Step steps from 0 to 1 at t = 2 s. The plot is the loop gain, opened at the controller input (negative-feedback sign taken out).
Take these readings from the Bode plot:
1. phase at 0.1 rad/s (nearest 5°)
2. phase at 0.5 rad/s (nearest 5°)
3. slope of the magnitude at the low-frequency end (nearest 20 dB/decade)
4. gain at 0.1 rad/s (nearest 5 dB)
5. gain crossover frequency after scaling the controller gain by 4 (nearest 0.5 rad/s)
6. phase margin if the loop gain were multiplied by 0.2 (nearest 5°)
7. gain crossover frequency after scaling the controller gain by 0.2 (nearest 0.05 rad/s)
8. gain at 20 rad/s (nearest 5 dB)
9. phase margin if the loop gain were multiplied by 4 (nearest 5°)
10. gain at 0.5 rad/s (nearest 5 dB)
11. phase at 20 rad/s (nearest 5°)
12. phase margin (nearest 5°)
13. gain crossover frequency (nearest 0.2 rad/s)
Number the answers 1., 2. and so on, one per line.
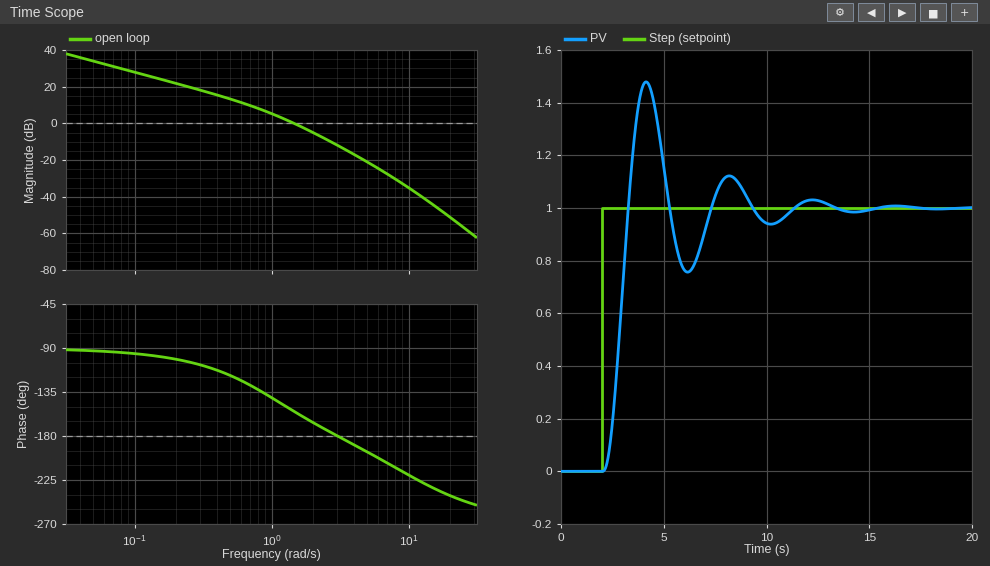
1. -95°
2. -120°
3. -20 dB/decade
4. 30 dB
5. 3.0 rad/s
6. 65°
7. 0.45 rad/s
8. -50 dB
9. 0°
10. 15 dB
11. -240°
12. 25°
13. 1.4 rad/s
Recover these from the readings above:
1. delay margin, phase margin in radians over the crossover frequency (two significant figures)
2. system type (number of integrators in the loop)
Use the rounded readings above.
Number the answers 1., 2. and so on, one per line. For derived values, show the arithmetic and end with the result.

1. 25 × π / 180 / 1.4 = 0.31 s
2. 1
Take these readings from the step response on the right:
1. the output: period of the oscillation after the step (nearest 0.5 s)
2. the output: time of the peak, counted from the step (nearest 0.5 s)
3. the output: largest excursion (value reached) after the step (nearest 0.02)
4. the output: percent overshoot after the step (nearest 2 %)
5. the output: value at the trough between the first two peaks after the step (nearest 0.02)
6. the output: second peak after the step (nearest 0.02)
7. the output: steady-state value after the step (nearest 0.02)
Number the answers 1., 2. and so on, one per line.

1. 4.0 s
2. 2.0 s
3. 1.48
4. 48 %
5. 0.76
6. 1.12
7. 1.00
